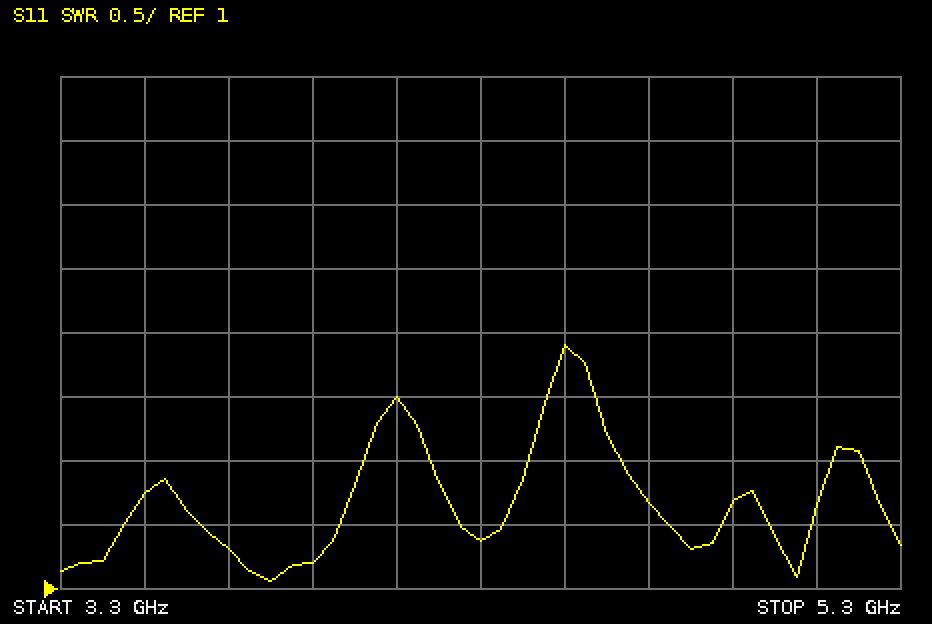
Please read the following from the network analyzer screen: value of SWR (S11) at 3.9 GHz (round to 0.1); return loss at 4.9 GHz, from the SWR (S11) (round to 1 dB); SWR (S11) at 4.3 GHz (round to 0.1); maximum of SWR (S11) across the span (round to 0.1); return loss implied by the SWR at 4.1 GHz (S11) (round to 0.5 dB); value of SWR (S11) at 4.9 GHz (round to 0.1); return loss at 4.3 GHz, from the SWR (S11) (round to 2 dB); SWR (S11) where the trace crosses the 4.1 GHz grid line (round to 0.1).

1.2
12 dB
1.4
2.9
7.5 dB
1.7
16 dB
2.5
